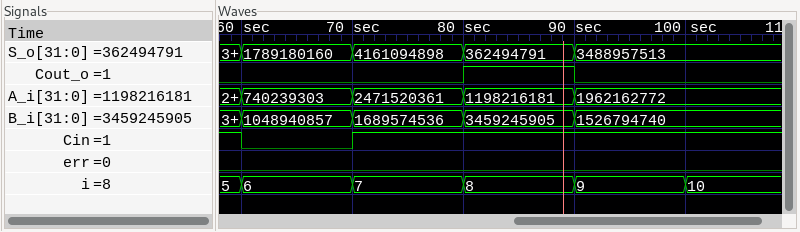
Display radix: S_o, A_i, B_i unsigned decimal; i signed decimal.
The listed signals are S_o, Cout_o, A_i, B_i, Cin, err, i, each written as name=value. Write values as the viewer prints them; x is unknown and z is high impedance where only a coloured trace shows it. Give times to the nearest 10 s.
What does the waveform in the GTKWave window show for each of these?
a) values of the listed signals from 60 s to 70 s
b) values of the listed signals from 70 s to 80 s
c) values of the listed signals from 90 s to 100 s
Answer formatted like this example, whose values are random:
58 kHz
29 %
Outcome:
S_o=1789180160, Cout_o=0, A_i=740239303, B_i=1048940857, Cin=0, err=0, i=6
S_o=4161094898, Cout_o=0, A_i=2471520361, B_i=1689574536, Cin=1, err=0, i=7
S_o=3488957513, Cout_o=0, A_i=1962162772, B_i=1526794740, Cin=1, err=0, i=9
